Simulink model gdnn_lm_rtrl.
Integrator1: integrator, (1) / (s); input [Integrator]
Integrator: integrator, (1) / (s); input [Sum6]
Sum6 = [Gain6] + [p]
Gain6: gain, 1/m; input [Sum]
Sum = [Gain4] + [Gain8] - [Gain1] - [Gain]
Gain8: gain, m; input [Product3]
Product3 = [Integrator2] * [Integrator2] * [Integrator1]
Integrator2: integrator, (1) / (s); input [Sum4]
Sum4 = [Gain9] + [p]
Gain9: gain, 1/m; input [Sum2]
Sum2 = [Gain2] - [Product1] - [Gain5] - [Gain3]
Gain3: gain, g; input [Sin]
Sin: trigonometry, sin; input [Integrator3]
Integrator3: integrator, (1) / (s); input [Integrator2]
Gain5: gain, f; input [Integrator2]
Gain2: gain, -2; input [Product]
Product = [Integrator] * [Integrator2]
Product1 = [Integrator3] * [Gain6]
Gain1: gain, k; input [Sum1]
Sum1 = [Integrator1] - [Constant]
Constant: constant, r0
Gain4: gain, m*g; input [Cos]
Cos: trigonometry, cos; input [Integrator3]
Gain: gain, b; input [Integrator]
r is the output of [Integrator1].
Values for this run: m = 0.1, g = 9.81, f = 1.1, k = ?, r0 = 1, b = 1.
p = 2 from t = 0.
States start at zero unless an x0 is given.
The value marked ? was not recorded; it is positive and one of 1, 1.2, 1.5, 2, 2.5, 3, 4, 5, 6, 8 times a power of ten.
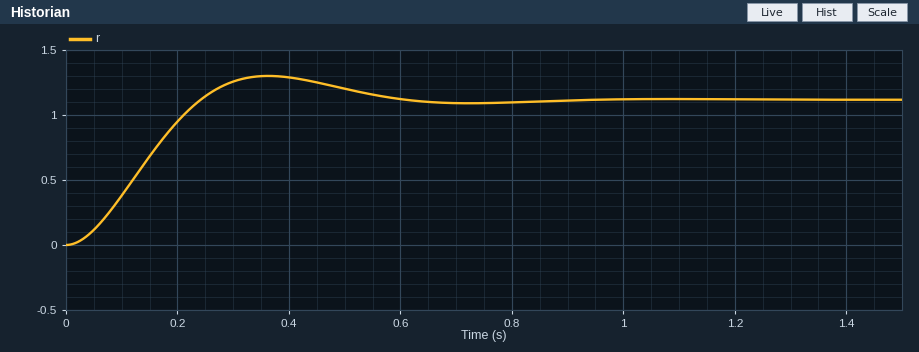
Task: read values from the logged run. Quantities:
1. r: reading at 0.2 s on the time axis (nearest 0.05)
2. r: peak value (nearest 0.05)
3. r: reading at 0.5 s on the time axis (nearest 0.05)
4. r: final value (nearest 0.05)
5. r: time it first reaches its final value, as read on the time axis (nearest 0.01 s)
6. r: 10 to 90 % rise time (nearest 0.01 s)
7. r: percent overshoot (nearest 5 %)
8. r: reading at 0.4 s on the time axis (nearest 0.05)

0.95
1.30
1.20
1.10
0.24 s
0.16 s
15 %
1.30
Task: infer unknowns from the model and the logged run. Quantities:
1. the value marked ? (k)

10
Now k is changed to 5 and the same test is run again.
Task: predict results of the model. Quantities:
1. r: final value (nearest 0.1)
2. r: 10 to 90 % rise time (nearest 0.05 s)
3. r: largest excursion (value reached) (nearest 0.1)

1.2
0.30 s
1.3
